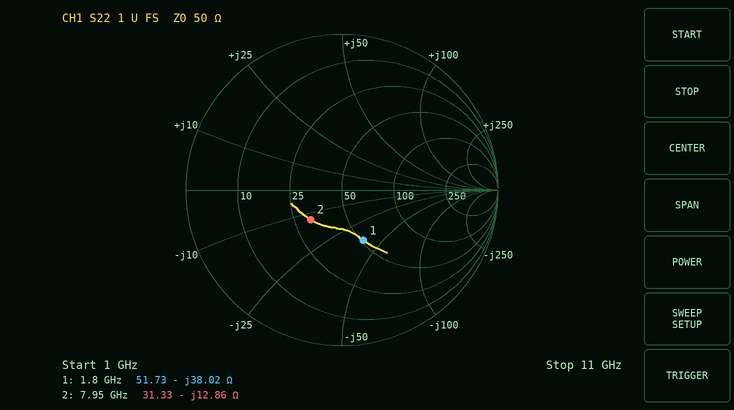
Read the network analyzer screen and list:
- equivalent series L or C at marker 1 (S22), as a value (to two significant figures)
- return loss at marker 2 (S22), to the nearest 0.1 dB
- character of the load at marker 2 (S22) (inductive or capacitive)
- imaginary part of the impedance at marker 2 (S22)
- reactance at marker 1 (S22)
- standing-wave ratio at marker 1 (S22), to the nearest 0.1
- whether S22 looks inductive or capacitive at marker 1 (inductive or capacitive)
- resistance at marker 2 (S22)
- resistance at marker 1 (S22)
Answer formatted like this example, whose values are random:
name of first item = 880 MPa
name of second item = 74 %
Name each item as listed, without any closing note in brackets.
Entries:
equivalent series L or C at marker 1 (S22), as a value = 2.3 pF
return loss at marker 2 (S22), to the nearest 0.1 dB = 11.2 dB
character of the load at marker 2 (S22) = capacitive
imaginary part of the impedance at marker 2 = -12.86 Ω
reactance at marker 1 = -38.02 Ω
standing-wave ratio at marker 1 (S22), to the nearest 0.1 = 2.1
whether S22 looks inductive or capacitive at marker 1 = capacitive
resistance at marker 2 = 31.33 Ω
resistance at marker 1 = 51.73 Ω
